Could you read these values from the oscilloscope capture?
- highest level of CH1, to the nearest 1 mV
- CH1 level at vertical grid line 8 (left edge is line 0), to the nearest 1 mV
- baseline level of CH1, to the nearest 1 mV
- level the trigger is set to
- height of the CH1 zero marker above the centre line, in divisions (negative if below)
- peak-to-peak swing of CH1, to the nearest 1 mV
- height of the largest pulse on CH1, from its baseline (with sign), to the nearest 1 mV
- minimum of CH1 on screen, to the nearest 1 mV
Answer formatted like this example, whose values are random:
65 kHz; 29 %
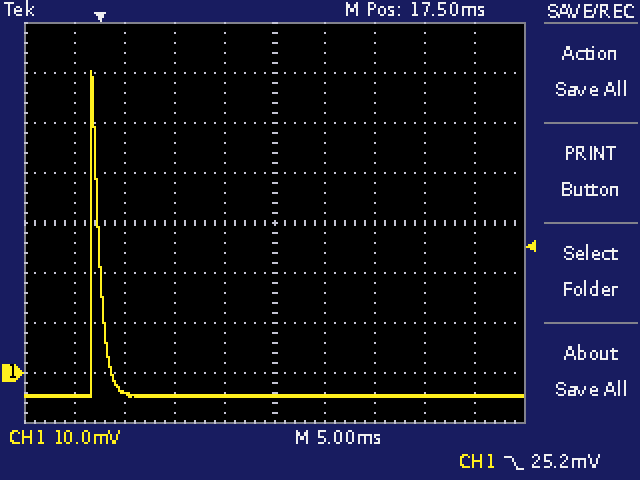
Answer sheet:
60 mV; -5 mV; -5 mV; 25.2 mV; -3.0 div; 65 mV; +65 mV; -5 mV
